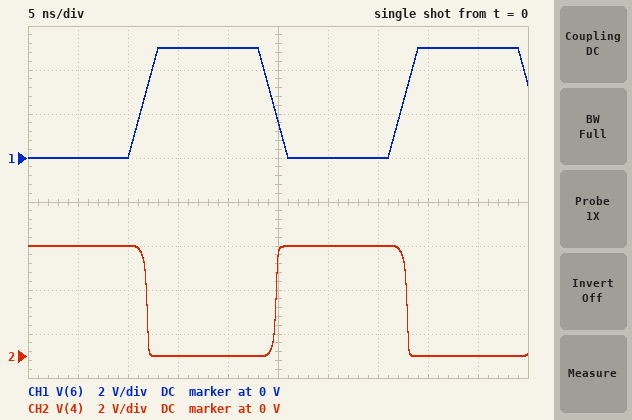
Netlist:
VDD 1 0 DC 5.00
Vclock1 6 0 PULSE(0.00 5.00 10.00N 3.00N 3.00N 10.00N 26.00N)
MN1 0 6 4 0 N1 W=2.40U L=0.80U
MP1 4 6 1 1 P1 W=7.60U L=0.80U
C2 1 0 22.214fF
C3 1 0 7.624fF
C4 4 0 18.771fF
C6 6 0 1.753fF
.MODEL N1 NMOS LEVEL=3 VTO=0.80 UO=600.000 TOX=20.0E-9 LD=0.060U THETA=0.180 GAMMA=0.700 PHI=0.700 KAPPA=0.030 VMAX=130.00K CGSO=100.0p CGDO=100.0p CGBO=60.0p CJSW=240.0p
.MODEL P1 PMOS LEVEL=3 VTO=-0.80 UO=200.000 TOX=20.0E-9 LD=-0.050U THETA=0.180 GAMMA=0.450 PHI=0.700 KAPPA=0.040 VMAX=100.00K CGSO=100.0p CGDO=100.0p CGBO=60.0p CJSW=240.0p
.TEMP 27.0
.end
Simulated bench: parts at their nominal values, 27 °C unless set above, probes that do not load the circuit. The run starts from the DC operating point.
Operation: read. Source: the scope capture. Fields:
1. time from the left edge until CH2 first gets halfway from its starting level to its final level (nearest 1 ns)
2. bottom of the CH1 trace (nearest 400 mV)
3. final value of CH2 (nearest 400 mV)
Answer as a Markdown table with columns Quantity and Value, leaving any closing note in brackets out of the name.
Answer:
| Quantity | Value |
|---|---|
| time from the left edge until CH2 first gets halfway from its starting level to its final level | 12 ns |
| bottom of the CH1 trace | 0 V |
| final value of CH2 | 0 V |
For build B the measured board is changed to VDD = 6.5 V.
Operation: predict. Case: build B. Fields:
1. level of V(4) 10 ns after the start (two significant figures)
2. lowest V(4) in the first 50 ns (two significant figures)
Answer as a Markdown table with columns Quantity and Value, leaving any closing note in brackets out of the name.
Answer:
| Quantity | Value |
|---|---|
| level of V(4) 10 ns after the start | 6.5 V |
| lowest V(4) in the first 50 ns | 58 mV |
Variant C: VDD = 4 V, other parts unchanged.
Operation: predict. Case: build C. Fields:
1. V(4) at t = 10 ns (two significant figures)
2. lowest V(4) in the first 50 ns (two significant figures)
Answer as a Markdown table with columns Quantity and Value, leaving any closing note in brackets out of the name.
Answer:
| Quantity | Value |
|---|---|
| V(4) at t = 10 ns | 4.0 V |
| lowest V(4) in the first 50 ns | -6.5 mV |
